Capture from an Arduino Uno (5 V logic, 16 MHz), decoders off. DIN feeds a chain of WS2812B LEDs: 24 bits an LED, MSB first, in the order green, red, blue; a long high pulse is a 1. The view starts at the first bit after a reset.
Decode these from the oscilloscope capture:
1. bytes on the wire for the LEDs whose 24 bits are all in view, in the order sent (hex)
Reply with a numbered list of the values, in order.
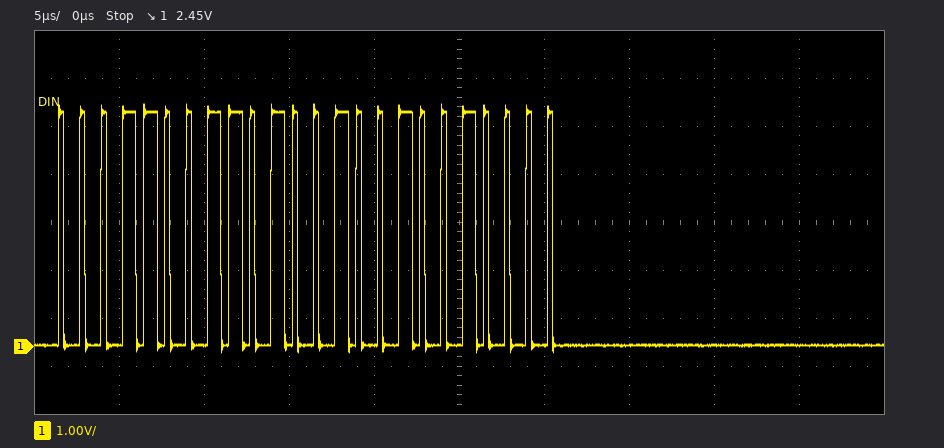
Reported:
1. 19 A4 90
